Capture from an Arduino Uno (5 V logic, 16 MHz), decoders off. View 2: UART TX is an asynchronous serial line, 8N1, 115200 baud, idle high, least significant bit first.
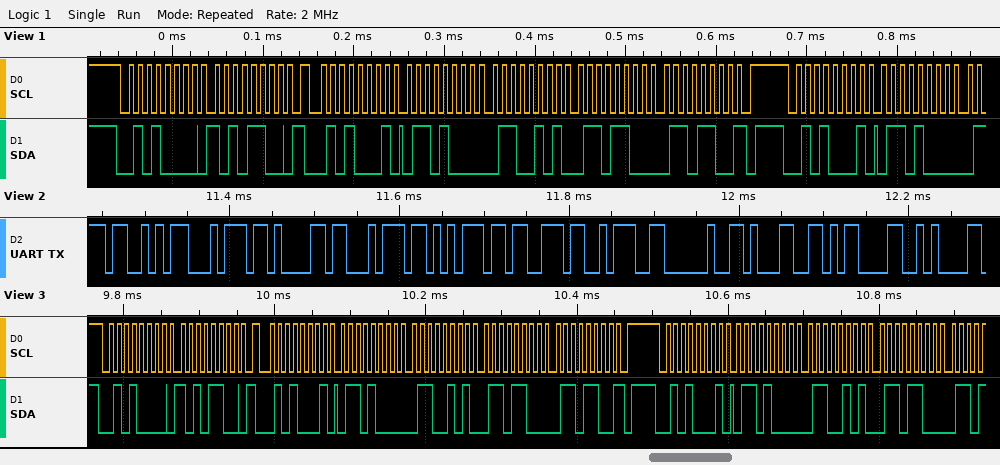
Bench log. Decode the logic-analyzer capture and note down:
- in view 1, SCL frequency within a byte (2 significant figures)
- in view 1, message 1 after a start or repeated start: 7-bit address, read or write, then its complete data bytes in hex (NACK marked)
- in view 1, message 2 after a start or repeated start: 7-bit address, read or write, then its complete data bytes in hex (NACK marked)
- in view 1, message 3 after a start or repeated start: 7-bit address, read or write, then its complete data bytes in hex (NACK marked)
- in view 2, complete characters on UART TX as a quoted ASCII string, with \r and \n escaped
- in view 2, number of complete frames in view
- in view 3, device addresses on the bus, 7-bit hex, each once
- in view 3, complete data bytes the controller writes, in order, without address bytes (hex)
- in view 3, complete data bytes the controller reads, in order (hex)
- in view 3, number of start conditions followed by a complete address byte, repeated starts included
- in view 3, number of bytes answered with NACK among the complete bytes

100 kHz
0x28 write: AC
0x28 read: 68 65 6C 6C NACK
0x28 read: 68
"Status: 1\r\n"
11
0x28
AC
68 65 6C 6C 68 65 6C
3
1
